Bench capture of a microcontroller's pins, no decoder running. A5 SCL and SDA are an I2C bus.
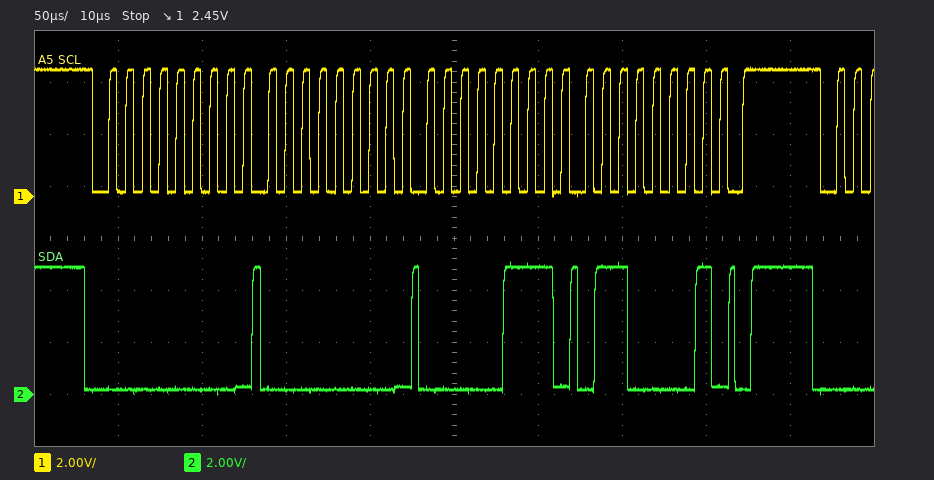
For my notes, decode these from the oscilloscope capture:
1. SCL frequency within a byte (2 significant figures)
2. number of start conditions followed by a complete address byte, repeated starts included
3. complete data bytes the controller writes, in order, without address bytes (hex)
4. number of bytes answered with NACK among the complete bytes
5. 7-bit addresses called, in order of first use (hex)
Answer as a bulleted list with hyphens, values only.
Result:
- 100 kHz
- 1
- 00 07 61
- 0
- 0x00
